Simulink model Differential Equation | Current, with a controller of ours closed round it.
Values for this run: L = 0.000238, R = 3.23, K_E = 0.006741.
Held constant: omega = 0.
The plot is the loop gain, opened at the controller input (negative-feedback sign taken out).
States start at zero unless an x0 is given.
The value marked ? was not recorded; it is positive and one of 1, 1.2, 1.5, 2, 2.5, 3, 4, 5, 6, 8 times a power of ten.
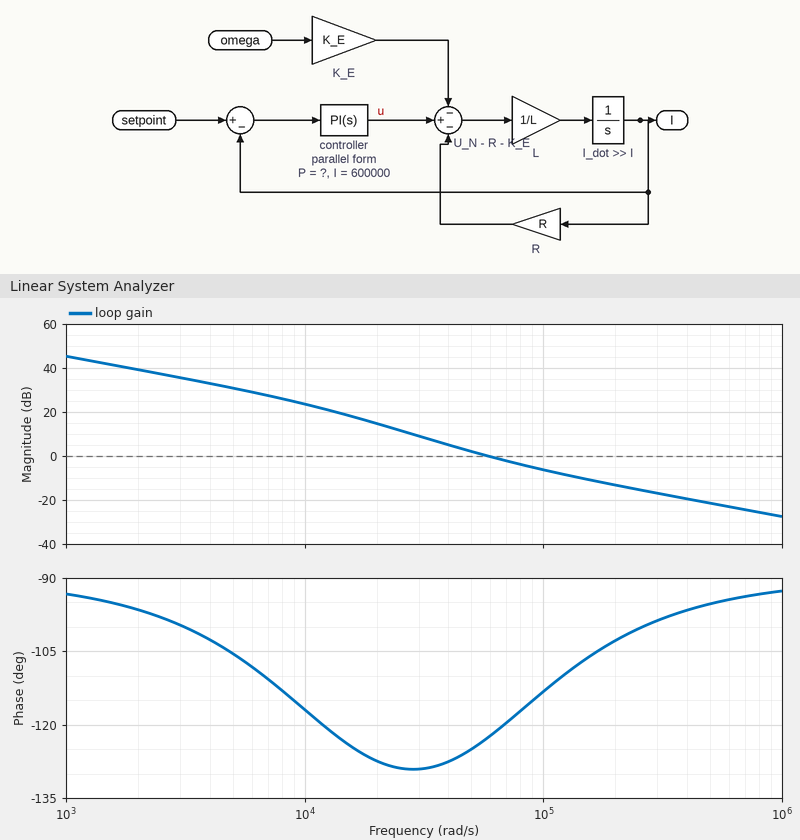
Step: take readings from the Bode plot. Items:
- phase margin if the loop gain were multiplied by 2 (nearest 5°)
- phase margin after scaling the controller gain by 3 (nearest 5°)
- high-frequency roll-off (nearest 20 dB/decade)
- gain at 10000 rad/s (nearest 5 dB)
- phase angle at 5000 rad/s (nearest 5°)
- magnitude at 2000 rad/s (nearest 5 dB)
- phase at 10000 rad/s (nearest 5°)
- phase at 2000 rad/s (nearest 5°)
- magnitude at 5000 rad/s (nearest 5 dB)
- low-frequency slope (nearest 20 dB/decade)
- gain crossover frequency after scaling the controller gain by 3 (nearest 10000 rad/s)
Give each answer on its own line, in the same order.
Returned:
65°
70°
-20 dB/decade
25 dB
-105°
40 dB
-115°
-95°
30 dB
-20 dB/decade
140000 rad/s
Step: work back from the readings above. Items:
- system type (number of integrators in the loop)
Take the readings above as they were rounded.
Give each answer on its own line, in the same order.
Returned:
1
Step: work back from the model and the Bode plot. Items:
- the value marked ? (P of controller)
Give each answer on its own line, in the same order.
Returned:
10
